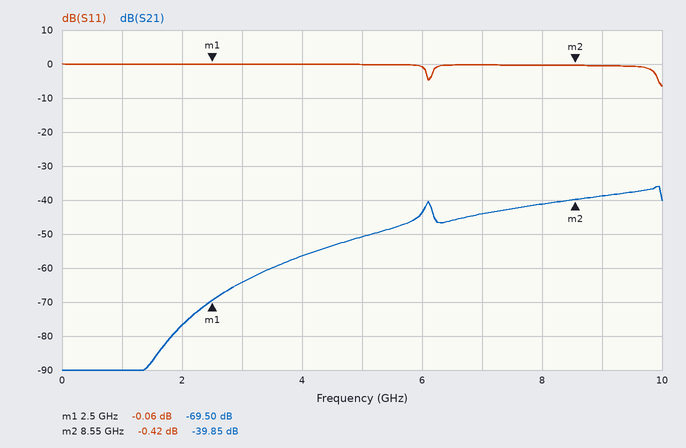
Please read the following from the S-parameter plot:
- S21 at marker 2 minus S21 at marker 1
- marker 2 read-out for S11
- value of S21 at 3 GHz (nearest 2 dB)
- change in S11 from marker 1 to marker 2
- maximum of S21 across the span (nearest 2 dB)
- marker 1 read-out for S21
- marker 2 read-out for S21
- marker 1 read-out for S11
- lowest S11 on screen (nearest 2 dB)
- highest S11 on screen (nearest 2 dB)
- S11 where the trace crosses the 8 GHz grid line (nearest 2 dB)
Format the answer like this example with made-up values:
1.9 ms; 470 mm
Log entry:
29.65 dB; -0.42 dB; -64 dB; -0.36 dB; -36 dB; -69.50 dB; -39.85 dB; -0.06 dB; -6 dB; 0 dB; 0 dB
